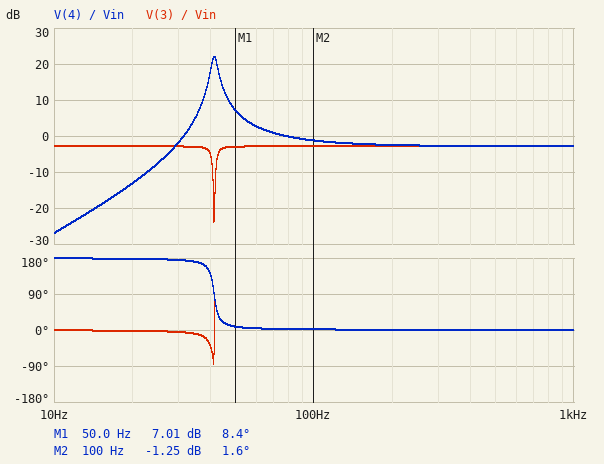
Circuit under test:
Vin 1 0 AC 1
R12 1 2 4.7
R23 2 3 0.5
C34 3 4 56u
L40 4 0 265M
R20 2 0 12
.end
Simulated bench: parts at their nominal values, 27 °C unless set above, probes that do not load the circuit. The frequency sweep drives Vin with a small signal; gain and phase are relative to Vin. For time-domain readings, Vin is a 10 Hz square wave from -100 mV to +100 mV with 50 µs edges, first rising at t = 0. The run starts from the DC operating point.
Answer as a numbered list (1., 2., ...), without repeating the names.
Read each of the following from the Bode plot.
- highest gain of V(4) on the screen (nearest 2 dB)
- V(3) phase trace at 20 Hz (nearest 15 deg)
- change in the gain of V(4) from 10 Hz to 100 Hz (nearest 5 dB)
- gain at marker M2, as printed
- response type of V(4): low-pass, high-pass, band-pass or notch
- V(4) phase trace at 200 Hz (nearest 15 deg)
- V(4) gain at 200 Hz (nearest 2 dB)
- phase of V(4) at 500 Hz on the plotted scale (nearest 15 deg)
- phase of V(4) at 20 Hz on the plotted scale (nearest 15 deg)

1. 22 dB
2. 0 deg
3. 25 dB
4. -1.25 dB
5. high-pass
6. 0 deg
7. -2 dB
8. 0 deg
9. 180 deg
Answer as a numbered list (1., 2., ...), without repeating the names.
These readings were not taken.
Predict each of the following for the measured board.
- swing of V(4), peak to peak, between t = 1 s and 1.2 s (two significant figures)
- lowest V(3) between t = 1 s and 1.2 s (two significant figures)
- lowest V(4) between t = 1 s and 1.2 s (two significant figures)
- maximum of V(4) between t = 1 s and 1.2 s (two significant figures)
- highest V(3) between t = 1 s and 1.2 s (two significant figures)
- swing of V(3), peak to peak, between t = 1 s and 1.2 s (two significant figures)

1. 170 mV
2. -76 mV
3. -86 mV
4. 86 mV
5. 76 mV
6. 150 mV
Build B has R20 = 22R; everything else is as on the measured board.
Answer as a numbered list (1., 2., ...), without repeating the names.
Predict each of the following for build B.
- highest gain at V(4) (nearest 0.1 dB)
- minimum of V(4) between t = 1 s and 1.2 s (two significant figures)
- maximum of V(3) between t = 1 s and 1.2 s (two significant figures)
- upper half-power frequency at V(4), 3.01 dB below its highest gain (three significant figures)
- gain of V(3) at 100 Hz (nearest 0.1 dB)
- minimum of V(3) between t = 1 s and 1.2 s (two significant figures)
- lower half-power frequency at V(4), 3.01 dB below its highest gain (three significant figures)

1. 22.3 dB
2. -100 mV
3. 88 mV
4. 42.7 Hz
5. -1.7 dB
6. -88 mV
7. 40.1 Hz
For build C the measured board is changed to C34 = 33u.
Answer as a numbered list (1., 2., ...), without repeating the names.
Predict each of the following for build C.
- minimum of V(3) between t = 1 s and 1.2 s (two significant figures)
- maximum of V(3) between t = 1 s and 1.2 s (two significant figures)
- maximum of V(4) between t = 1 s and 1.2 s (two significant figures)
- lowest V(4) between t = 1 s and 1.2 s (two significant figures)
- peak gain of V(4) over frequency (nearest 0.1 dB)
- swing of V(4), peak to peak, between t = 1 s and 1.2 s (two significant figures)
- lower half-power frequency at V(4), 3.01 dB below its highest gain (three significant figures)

1. -78 mV
2. 78 mV
3. 140 mV
4. -140 mV
5. 24.4 dB
6. 280 mV
7. 52.7 Hz
